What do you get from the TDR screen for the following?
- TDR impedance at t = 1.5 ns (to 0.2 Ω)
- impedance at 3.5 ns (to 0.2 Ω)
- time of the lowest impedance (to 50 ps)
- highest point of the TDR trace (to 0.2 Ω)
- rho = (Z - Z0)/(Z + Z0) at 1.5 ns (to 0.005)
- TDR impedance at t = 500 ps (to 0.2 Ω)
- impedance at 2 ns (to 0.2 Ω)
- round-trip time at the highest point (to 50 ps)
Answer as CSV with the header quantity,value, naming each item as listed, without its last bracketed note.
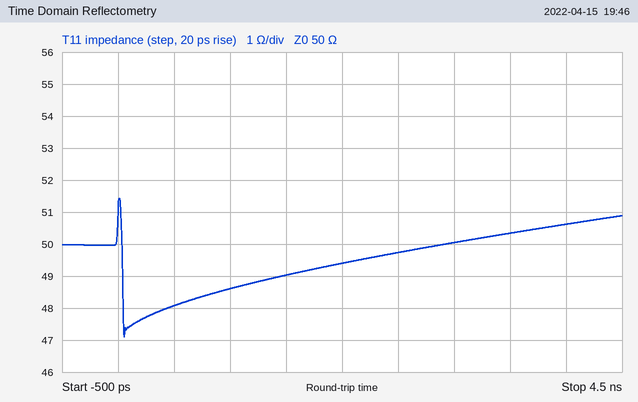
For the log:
quantity,value
TDR impedance at t = 1.5 ns,49.0 Ω
impedance at 3.5 ns,50.4 Ω
time of the lowest impedance,50 ps
highest point of the TDR trace,51.4 Ω
rho = (Z - Z0)/(Z + Z0) at 1.5 ns,-0.010
TDR impedance at t = 500 ps,48.0 Ω
impedance at 2 ns,49.4 Ω
round-trip time at the highest point,0 ps
